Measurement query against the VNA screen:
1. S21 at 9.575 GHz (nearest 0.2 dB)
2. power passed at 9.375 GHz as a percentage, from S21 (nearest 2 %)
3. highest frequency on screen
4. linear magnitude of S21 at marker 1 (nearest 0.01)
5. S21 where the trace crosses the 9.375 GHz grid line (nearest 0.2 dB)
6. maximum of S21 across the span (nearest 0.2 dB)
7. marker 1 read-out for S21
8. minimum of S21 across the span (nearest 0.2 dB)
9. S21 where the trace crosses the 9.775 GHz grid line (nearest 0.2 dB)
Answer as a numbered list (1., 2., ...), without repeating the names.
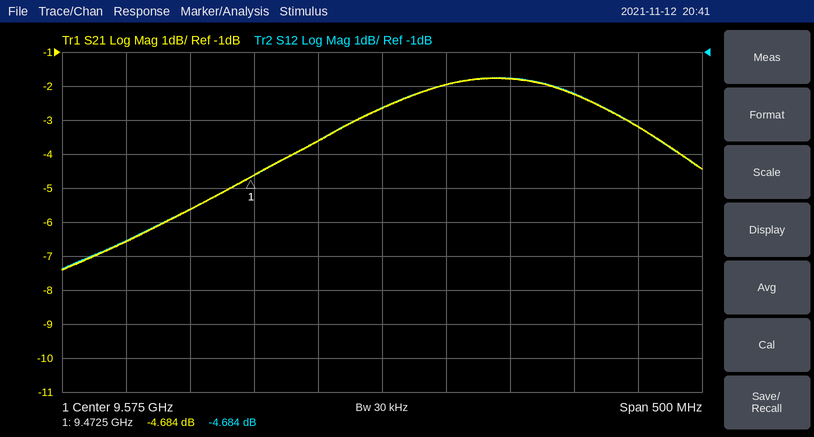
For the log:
1. -2.6 dB
2. 22 %
3. 9.825 GHz
4. 0.58
5. -6.6 dB
6. -1.8 dB
7. -4.684 dB
8. -7.4 dB
9. -3.2 dB
